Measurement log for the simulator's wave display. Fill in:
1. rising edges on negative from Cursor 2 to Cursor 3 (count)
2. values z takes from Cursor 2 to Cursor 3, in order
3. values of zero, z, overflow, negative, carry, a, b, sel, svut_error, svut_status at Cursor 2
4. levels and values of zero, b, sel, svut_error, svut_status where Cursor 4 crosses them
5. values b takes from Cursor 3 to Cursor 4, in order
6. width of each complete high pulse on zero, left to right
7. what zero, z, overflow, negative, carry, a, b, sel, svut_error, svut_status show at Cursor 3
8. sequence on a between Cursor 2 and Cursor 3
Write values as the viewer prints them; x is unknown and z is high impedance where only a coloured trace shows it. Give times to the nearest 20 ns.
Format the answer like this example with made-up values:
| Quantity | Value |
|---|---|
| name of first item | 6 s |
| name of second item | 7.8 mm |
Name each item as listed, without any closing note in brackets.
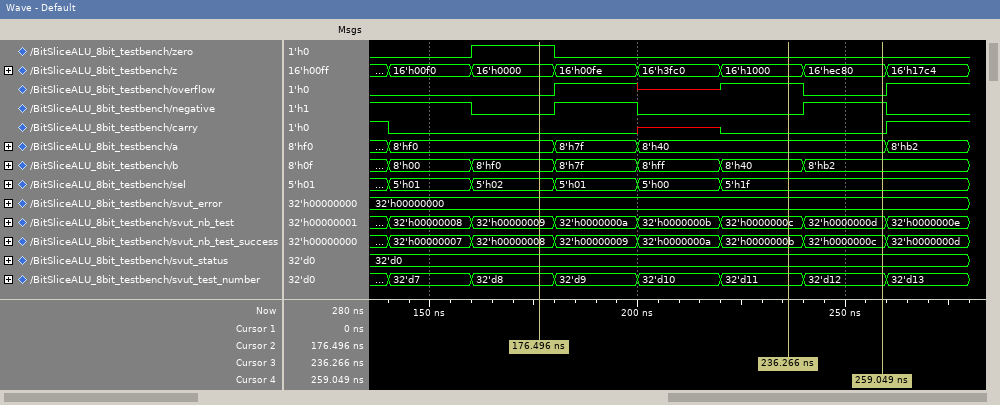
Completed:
| Quantity | Value |
|---|---|
| rising edges on negative from Cursor 2 to Cursor 3 | 1 |
| values z takes from Cursor 2 to Cursor 3, in order | 16'h0000, 16'h00fe, 16'h3fc0, 16'h1000 |
| values of zero, z, overflow, negative, carry, a, b, sel, svut_error, svut_status at Cursor 2 | zero=1, z=16'h0000, overflow=0, negative=0, carry=0, a=8'hf0, b=8'hf0, sel=5'h02, svut_error=32'h00000000, svut_status=32'd0 |
| levels and values of zero, b, sel, svut_error, svut_status where Cursor 4 crosses them | zero=0, b=8'hb2, sel=5'h1f, svut_error=32'h00000000, svut_status=32'd0 |
| values b takes from Cursor 3 to Cursor 4, in order | 8'h40, 8'hb2 |
| width of each complete high pulse on zero, left to right | 20 ns |
| what zero, z, overflow, negative, carry, a, b, sel, svut_error, svut_status show at Cursor 3 | zero=0, z=16'h1000, overflow=1, negative=0, carry=0, a=8'h40, b=8'h40, sel=5'h1f, svut_error=32'h00000000, svut_status=32'd0 |
| sequence on a between Cursor 2 and Cursor 3 | 8'hf0, 8'h7f, 8'h40 |
